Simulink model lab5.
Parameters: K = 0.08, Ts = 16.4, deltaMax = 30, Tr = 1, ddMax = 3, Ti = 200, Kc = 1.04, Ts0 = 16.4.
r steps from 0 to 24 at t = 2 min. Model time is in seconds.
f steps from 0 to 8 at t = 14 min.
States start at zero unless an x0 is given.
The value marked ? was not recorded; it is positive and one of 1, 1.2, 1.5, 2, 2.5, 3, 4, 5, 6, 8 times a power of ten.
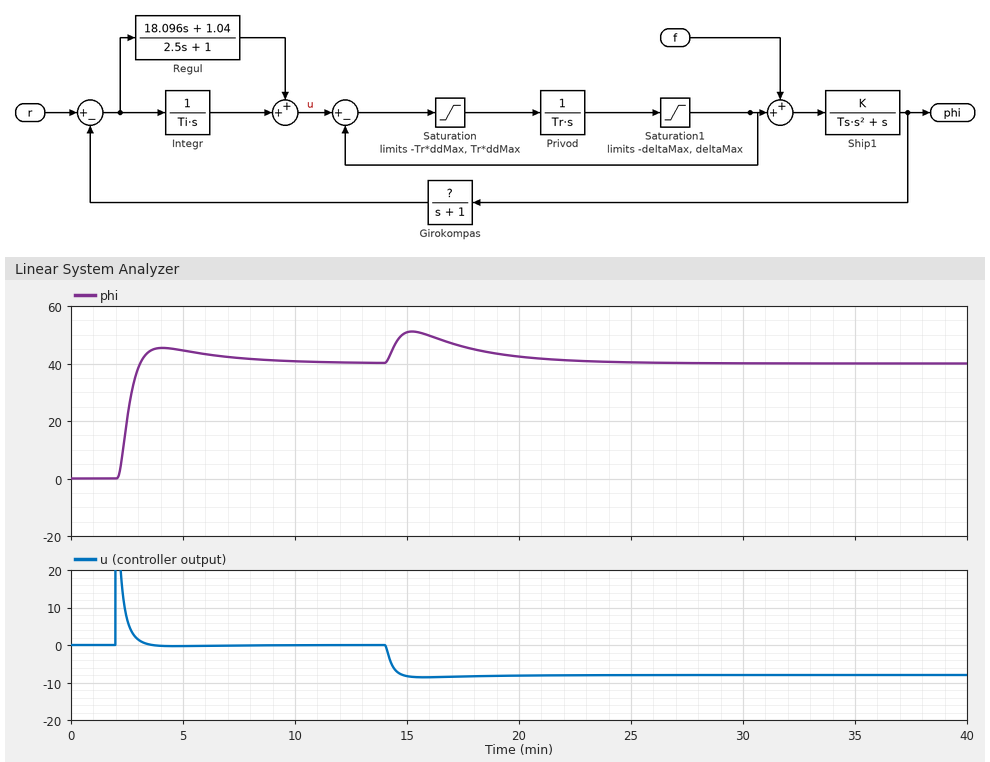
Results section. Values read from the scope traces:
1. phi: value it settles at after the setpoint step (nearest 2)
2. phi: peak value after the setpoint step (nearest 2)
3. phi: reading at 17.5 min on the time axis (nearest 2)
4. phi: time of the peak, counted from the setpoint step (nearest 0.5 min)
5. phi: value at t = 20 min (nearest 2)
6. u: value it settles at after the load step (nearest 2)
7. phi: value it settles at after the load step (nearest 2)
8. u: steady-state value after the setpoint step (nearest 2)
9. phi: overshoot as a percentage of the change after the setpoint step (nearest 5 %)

40
46
46
2.0 min
42
-8
40
0
15 %
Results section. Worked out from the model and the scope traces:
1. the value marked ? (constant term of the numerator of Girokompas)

0.6
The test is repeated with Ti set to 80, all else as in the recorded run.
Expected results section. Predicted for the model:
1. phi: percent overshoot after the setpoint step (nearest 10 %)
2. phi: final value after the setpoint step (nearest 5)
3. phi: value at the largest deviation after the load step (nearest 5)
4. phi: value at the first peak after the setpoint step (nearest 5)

30 %
40
50
50
